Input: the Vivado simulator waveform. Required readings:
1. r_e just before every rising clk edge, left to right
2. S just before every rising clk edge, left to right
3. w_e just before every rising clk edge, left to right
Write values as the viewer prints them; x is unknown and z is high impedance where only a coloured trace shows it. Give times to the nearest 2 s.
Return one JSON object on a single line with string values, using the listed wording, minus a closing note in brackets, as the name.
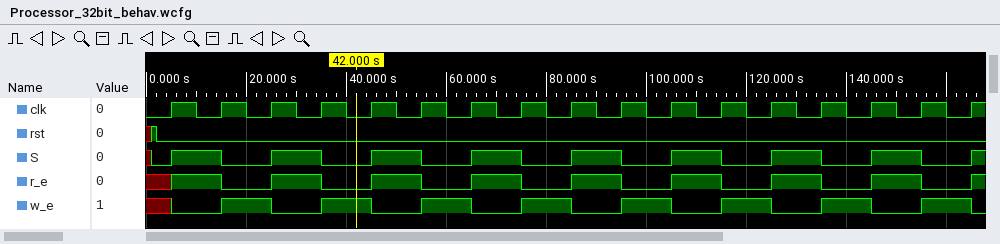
{"r_e just before every rising clk edge, left to right": "x 1 0 1 0 1 0 1 0 1 0 1 0 1 0 1 0", "S just before every rising clk edge, left to right": "0 1 0 1 0 1 0 1 0 1 0 1 0 1 0 1 0", "w_e just before every rising clk edge, left to right": "x 0 1 0 1 0 1 0 1 0 1 0 1 0 1 0 1"}
